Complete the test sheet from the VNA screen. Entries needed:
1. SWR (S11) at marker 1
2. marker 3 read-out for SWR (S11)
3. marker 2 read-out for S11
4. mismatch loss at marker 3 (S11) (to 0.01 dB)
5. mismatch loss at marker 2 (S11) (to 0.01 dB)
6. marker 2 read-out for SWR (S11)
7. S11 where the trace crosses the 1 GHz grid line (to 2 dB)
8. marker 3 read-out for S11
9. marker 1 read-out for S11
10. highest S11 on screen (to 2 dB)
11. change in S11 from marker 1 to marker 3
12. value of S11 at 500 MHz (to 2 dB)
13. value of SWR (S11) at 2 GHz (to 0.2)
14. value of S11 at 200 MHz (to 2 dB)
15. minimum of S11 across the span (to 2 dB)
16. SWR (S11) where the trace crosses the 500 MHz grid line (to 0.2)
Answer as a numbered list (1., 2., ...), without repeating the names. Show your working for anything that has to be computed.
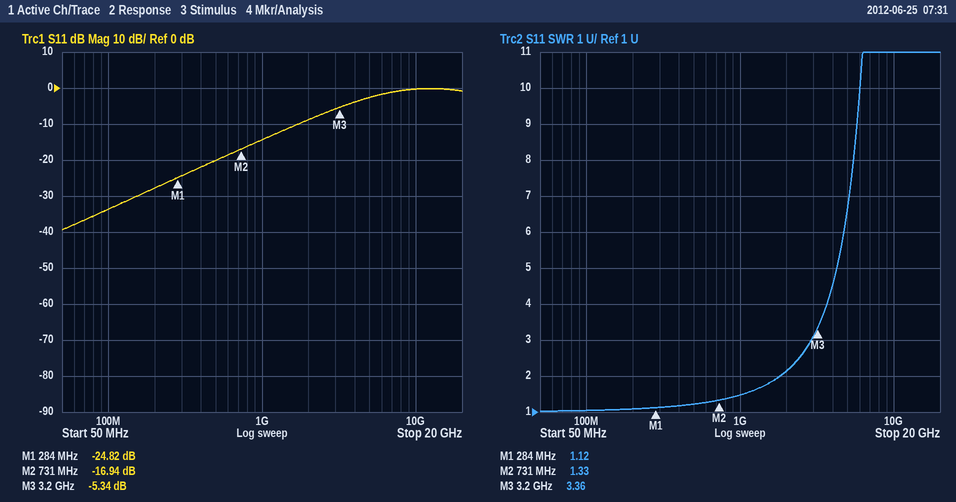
1. 1.12
2. 3.36
3. -16.94 dB
4. −10 log10(1 − 10^(-5.34/10)) ≈ 1.50 dB
5. −10 log10(1 − 10^(-16.94/10)) ≈ 0.09 dB
6. 1.33
7. -14 dB
8. -5.34 dB
9. -24.82 dB
10. 0 dB
11. -5.34 − (-24.82) = 19.48 dB
12. -20 dB
13. 2.2
14. -28 dB
15. -40 dB
16. 1.2
